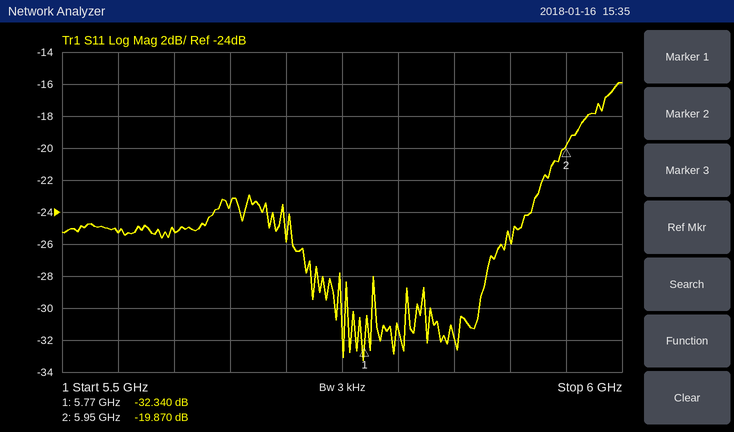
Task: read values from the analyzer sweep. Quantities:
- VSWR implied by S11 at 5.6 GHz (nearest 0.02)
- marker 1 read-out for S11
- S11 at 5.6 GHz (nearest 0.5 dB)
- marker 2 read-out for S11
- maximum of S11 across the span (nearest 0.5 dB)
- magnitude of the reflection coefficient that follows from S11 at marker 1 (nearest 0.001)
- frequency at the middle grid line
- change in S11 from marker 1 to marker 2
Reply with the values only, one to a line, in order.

1.12
-32.340 dB
-25.0 dB
-19.870 dB
-16.0 dB
0.024
5.75 GHz
12.470 dB
